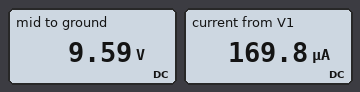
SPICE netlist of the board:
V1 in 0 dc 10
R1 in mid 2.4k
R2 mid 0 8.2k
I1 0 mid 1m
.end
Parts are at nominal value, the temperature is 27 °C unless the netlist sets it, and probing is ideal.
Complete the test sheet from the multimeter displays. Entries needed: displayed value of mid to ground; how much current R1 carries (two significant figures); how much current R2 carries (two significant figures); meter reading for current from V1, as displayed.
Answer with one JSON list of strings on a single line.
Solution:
["9.59 V", "170 µA", "1.2 mA", "169.8 µA"]
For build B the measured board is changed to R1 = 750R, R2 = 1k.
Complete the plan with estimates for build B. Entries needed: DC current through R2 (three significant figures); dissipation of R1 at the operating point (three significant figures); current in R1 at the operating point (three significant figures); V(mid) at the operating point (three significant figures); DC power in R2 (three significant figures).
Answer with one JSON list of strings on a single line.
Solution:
["6.14 mA", "19.8 mW", "5.14 mA", "6.14 V", "37.7 mW"]
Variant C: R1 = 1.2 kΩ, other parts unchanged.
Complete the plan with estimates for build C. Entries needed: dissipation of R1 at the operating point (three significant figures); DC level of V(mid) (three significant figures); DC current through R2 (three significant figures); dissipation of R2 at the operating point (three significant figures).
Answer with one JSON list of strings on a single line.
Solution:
["44.0 µW", "9.77 V", "1.19 mA", "11.6 mW"]
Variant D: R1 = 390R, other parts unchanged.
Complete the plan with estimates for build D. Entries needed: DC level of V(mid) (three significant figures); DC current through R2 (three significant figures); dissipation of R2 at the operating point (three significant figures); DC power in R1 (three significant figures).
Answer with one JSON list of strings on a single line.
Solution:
["9.92 V", "1.21 mA", "12.0 mW", "17.1 µW"]
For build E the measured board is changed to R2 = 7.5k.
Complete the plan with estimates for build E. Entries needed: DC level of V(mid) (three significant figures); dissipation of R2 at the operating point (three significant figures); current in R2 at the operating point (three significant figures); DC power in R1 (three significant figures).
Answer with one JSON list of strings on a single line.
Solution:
["9.39 V", "11.8 mW", "1.25 mA", "153 µW"]
